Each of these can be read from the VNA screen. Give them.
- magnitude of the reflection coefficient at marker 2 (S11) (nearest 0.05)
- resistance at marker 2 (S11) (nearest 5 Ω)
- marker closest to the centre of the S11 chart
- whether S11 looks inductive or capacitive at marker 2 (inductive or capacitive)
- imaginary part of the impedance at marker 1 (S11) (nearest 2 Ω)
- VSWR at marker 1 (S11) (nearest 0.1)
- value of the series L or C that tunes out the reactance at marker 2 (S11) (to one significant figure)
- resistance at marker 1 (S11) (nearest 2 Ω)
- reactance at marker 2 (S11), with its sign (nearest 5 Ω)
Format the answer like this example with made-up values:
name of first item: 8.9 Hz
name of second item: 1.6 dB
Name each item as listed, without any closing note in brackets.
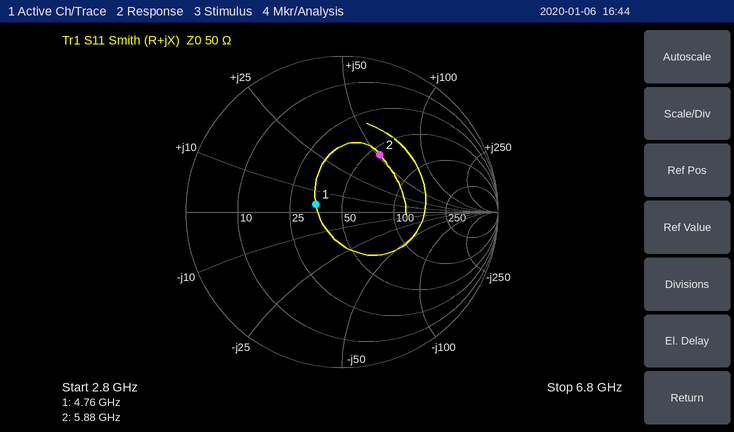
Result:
magnitude of the reflection coefficient at marker 2 (S11): 0.45
resistance at marker 2 (S11): 55 Ω
marker closest to the centre of the S11 chart: marker 1
whether S11 looks inductive or capacitive at marker 2: inductive
imaginary part of the impedance at marker 1 (S11): +4 Ω
VSWR at marker 1 (S11): 1.4
value of the series L or C that tunes out the reactance at marker 2 (S11): 500 fF
resistance at marker 1 (S11): 36 Ω
reactance at marker 2 (S11), with its sign: +50 Ω
